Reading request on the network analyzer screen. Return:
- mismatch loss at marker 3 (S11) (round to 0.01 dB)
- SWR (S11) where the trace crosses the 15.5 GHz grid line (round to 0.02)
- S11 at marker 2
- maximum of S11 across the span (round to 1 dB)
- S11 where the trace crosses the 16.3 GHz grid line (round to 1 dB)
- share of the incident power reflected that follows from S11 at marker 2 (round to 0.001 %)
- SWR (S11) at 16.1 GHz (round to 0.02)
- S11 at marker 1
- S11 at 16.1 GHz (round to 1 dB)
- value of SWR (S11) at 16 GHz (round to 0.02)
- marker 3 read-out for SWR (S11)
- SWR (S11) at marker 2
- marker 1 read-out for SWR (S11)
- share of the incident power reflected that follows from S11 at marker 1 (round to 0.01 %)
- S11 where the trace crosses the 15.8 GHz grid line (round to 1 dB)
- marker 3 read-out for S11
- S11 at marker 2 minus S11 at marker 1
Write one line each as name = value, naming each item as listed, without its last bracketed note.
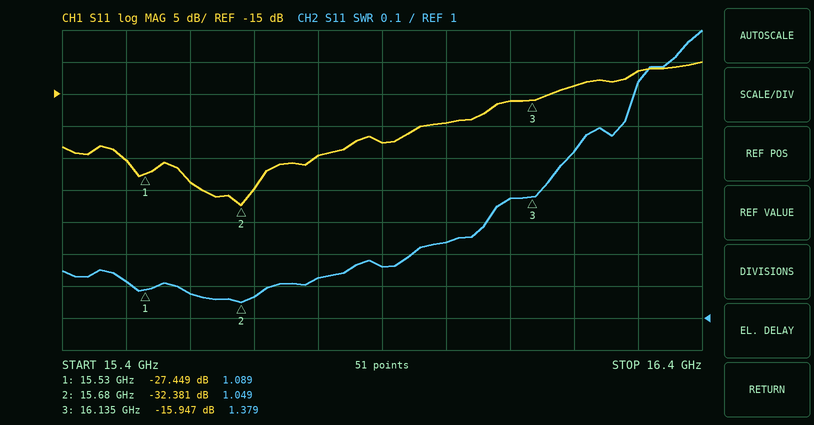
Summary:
mismatch loss at marker 3 (S11) = 0.11 dB
SWR (S11) where the trace crosses the 15.5 GHz grid line = 1.12
S11 at marker 2 = -32.381 dB
maximum of S11 across the span = -10 dB
S11 where the trace crosses the 16.3 GHz grid line = -11 dB
share of the incident power reflected that follows from S11 at marker 2 = 0.058 %
SWR (S11) at 16.1 GHz = 1.38
S11 at marker 1 = -27.449 dB
S11 at 16.1 GHz = -16 dB
value of SWR (S11) at 16 GHz = 1.24
marker 3 read-out for SWR = 1.379
SWR (S11) at marker 2 = 1.049
marker 1 read-out for SWR = 1.089
share of the incident power reflected that follows from S11 at marker 1 = 0.18 %
S11 where the trace crosses the 15.8 GHz grid line = -25 dB
marker 3 read-out for S11 = -15.947 dB
S11 at marker 2 minus S11 at marker 1 = -4.932 dB
